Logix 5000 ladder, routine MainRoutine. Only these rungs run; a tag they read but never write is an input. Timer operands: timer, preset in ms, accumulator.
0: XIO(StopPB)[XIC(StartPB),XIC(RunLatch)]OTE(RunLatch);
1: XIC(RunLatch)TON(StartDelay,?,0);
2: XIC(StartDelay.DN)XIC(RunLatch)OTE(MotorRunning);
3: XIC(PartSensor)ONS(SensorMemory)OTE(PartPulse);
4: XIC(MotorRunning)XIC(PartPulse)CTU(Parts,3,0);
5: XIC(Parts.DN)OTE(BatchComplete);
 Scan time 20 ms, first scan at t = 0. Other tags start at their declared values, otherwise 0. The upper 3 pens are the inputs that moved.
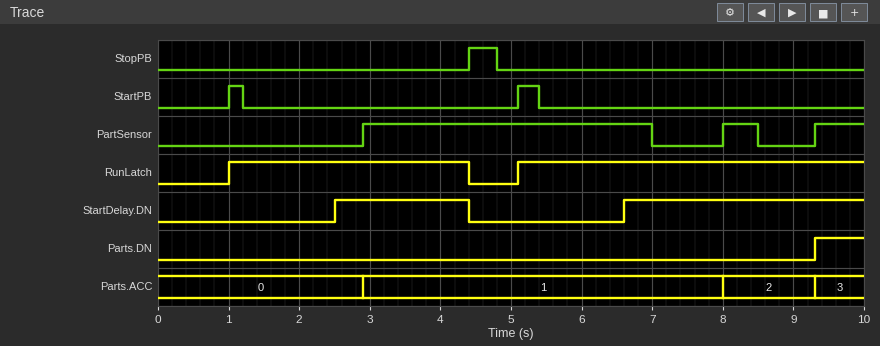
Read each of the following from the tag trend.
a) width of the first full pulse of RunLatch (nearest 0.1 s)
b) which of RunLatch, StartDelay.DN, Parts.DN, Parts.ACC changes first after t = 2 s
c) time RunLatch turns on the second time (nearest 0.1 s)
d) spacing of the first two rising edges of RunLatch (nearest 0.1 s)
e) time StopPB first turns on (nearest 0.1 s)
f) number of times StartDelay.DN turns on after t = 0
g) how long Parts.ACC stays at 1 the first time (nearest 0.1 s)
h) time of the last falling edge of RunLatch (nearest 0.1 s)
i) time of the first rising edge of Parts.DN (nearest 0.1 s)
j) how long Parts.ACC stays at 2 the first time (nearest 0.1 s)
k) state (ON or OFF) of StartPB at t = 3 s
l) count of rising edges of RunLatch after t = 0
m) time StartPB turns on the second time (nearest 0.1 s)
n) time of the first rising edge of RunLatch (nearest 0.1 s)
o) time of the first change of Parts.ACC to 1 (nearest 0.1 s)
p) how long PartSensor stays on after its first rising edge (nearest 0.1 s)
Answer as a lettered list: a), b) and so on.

a) 3.4 s
b) StartDelay.DN
c) 5.1 s
d) 4.1 s
e) 4.4 s
f) 2
g) 5.1 s
h) 4.4 s
i) 9.3 s
j) 1.3 s
k) OFF
l) 2
m) 5.1 s
n) 1.0 s
o) 2.9 s
p) 4.1 s
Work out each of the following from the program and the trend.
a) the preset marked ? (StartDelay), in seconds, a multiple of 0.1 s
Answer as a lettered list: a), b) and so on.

a) 1.5 s
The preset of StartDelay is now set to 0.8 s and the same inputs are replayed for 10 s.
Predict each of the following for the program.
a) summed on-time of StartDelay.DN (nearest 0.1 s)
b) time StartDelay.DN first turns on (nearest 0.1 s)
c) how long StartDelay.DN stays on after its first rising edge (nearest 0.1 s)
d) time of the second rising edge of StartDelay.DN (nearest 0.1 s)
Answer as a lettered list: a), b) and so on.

a) 6.7 s
b) 1.8 s
c) 2.6 s
d) 5.9 s
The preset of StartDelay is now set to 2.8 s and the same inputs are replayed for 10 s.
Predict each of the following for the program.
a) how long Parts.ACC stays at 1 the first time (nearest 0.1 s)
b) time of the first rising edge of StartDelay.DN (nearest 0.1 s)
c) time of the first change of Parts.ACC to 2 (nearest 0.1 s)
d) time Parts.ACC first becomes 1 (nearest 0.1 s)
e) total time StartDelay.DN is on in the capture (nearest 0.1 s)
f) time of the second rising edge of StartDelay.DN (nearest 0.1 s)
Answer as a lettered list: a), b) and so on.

a) 1.3 s
b) 3.8 s
c) 9.3 s
d) 8.0 s
e) 2.7 s
f) 7.9 s
